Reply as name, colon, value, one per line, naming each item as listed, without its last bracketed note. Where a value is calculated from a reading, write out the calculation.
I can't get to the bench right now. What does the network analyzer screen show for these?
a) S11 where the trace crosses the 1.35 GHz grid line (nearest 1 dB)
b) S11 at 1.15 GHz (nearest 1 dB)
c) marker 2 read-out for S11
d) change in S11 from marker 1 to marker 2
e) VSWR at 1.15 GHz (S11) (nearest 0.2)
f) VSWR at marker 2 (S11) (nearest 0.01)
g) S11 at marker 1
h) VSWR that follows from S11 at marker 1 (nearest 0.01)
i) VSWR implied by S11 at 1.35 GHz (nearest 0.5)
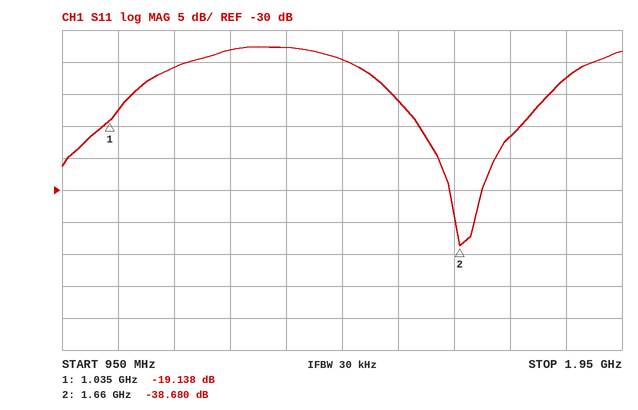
S11 where the trace crosses the 1.35 GHz grid line: -8 dB
S11 at 1.15 GHz: -11 dB
marker 2 read-out for S11: -38.680 dB
change in S11 from marker 1 to marker 2: -38.68 − (-19.138) = -19.542 dB
VSWR at 1.15 GHz (S11): |Γ| = 10^(-11/20) = 0.2818; VSWR = (1 + 0.2818)/(1 − 0.2818) ≈ 1.8
VSWR at marker 2 (S11): (1 + 0.0116)/(1 − 0.0116) ≈ 1.02
S11 at marker 1: -19.138 dB
VSWR that follows from S11 at marker 1: (1 + 0.1104)/(1 − 0.1104) ≈ 1.25
VSWR implied by S11 at 1.35 GHz: |Γ| = 10^(-8/20) = 0.3981; VSWR = (1 + 0.3981)/(1 − 0.3981) ≈ 2.32, so 2.5 to the nearest 0.5
